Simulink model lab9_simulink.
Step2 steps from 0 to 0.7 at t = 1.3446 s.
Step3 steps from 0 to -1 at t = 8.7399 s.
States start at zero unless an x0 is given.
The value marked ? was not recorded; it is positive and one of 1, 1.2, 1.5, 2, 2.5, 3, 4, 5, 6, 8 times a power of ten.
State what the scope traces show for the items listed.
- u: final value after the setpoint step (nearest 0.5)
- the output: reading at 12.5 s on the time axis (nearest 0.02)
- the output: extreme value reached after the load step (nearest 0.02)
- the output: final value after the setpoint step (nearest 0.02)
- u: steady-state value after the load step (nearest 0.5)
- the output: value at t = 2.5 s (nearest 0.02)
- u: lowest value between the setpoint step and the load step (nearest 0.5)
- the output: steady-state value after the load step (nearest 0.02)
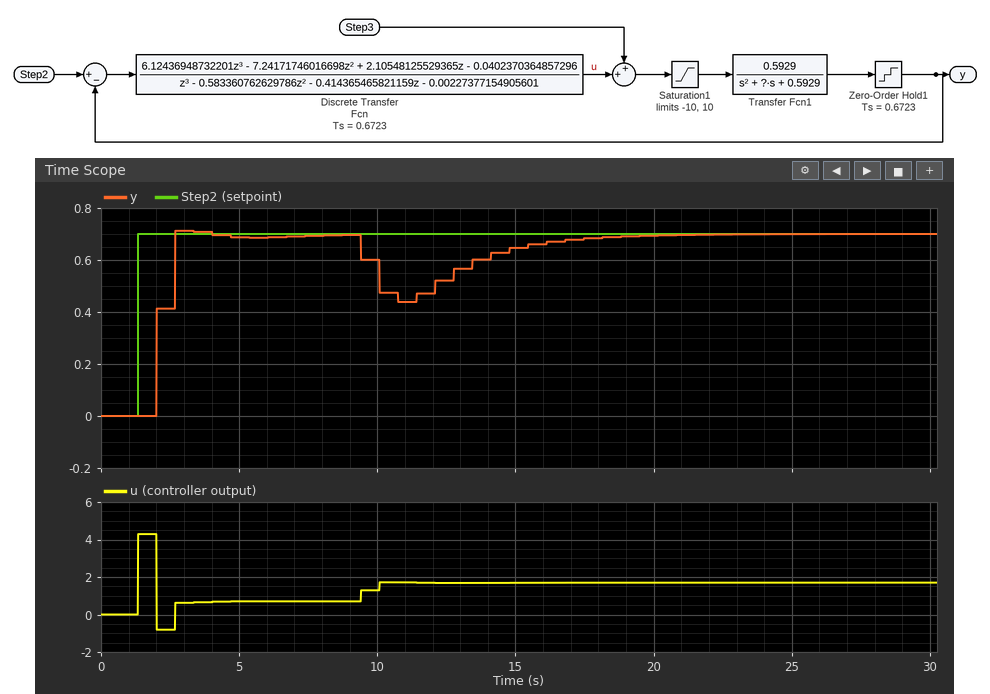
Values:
0.5
0.52
0.44
0.70
1.5
0.42
-1.0
0.70
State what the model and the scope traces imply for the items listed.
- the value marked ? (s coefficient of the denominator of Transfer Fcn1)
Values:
1.5
